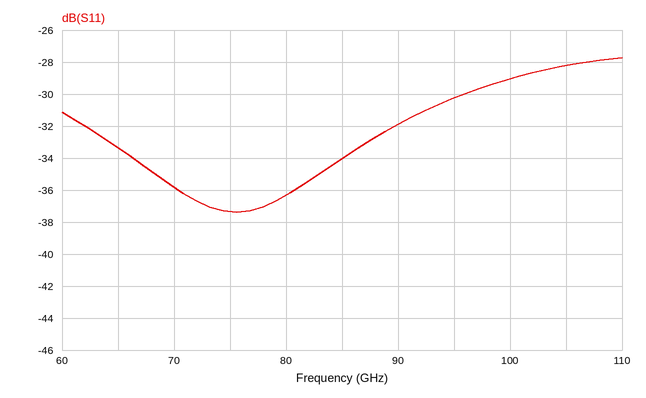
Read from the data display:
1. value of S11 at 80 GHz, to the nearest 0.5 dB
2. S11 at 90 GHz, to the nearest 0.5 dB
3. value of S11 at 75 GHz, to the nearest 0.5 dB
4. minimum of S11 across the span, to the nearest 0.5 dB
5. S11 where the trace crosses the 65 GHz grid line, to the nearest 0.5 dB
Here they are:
-36.5 dB
-32.0 dB
-37.5 dB
-37.5 dB
-33.5 dB
